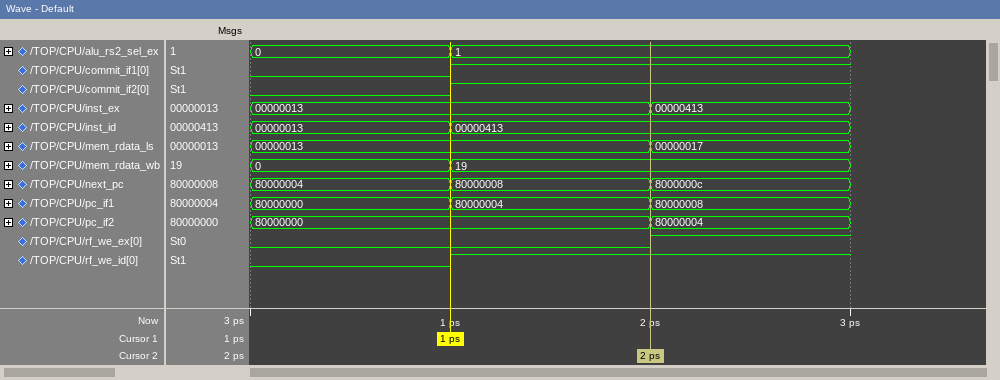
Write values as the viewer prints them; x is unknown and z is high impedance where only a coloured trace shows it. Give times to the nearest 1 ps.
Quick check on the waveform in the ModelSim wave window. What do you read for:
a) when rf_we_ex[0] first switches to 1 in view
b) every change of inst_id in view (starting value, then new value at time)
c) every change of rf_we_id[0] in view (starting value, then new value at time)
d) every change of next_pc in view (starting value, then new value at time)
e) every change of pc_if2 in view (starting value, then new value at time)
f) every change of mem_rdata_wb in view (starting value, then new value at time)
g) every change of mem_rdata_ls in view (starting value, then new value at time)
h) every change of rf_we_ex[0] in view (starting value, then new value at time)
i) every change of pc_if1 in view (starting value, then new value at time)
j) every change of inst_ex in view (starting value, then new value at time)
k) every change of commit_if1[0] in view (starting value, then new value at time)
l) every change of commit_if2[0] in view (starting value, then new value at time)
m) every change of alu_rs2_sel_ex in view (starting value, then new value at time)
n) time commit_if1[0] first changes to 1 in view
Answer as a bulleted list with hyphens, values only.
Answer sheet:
- 2 ps
- 00000013, 00000413 at 1 ps
- 0, 1 at 1 ps
- 80000004, 80000008 at 1 ps, 8000000c at 2 ps
- 80000000, 80000004 at 2 ps
- 0, 19 at 1 ps
- 00000013, 00000017 at 2 ps
- 0, 1 at 2 ps
- 80000000, 80000004 at 1 ps, 80000008 at 2 ps
- 00000013, 00000413 at 2 ps
- 0, 1 at 1 ps
- 0, 1 at 1 ps
- 0, 1 at 1 ps
- 1 ps
